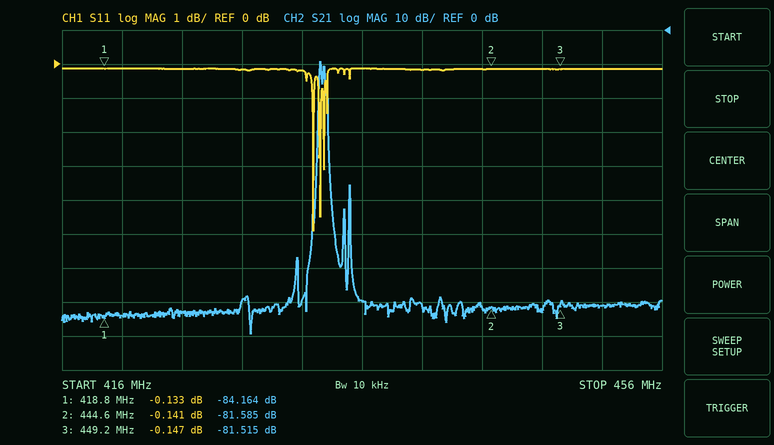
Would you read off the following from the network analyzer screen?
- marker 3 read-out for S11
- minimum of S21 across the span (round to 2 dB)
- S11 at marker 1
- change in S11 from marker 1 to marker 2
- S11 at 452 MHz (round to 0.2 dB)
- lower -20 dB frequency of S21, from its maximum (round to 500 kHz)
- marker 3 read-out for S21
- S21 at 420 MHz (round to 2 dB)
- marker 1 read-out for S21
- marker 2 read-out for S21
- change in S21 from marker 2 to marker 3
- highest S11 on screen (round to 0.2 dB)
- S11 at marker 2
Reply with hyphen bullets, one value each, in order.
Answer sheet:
- -0.147 dB
- -90 dB
- -0.133 dB
- -0.008 dB
- -0.2 dB
- 433.0 MHz
- -81.515 dB
- -84 dB
- -84.164 dB
- -81.585 dB
- 0.070 dB
- -0.2 dB
- -0.141 dB
